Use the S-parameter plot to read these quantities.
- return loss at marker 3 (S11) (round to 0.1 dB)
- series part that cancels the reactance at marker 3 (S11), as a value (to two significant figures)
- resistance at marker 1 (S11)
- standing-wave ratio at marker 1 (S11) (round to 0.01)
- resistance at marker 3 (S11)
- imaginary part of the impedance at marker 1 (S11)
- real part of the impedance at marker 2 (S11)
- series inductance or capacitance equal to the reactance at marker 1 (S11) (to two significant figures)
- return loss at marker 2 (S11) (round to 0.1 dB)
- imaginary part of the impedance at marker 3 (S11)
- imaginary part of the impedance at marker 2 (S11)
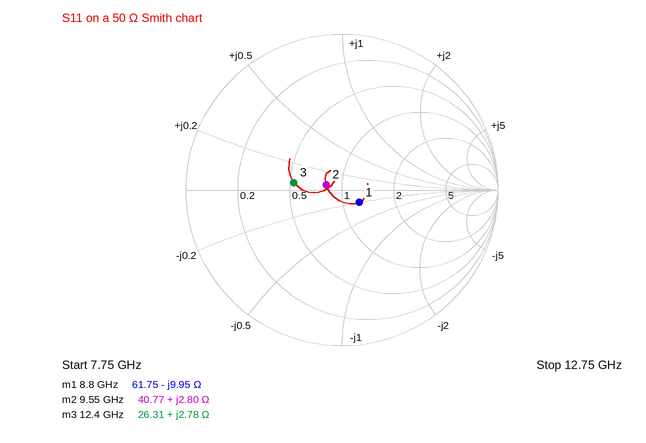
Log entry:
10.1 dB
4.6 pF
61.75 Ω
1.32
26.31 Ω
-9.95 Ω
40.77 Ω
1.8 pF
19.5 dB
+2.78 Ω
+2.80 Ω
